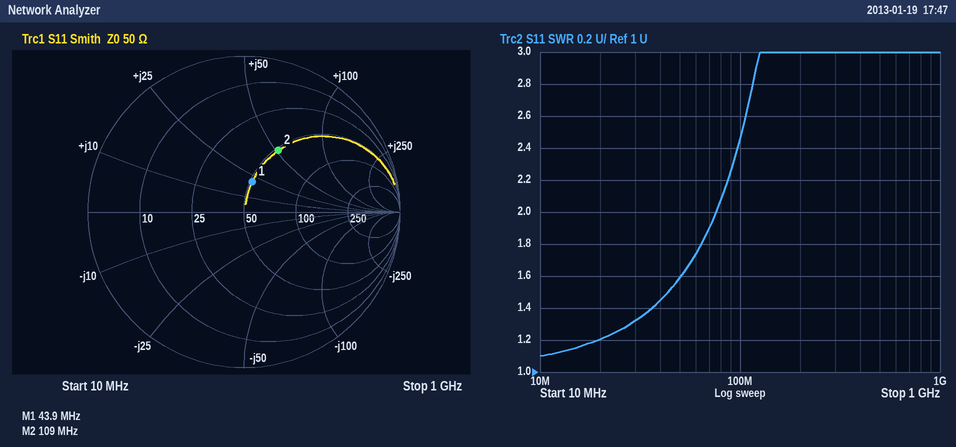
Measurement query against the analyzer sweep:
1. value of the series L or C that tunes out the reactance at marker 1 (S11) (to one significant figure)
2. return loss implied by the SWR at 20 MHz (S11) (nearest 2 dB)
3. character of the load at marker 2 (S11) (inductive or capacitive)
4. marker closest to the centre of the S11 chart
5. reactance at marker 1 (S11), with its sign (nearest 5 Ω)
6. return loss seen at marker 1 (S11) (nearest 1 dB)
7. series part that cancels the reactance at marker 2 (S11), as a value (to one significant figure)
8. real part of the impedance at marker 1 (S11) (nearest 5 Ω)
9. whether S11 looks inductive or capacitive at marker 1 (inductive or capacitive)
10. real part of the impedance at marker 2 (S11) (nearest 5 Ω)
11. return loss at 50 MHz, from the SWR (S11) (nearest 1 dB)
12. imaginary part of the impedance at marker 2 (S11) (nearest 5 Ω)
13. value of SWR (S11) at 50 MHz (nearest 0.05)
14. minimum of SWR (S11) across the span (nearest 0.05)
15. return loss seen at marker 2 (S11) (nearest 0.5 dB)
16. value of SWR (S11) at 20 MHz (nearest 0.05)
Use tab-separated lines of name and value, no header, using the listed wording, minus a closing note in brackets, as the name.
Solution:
value of the series L or C that tunes out the reactance at marker 1 (S11)	200 pF
return loss implied by the SWR at 20 MHz (S11)	20 dB
character of the load at marker 2 (S11)	inductive
marker closest to the centre of the S11 chart	marker 1
reactance at marker 1 (S11), with its sign	+20 Ω
return loss seen at marker 1 (S11)	14 dB
series part that cancels the reactance at marker 2 (S11), as a value	30 pF
real part of the impedance at marker 1 (S11)	50 Ω
whether S11 looks inductive or capacitive at marker 1	inductive
real part of the impedance at marker 2 (S11)	50 Ω
return loss at 50 MHz, from the SWR (S11)	13 dB
imaginary part of the impedance at marker 2 (S11)	+50 Ω
value of SWR (S11) at 50 MHz	1.60
minimum of SWR (S11) across the span	1.10
return loss seen at marker 2 (S11)	7.0 dB
value of SWR (S11) at 20 MHz	1.20
